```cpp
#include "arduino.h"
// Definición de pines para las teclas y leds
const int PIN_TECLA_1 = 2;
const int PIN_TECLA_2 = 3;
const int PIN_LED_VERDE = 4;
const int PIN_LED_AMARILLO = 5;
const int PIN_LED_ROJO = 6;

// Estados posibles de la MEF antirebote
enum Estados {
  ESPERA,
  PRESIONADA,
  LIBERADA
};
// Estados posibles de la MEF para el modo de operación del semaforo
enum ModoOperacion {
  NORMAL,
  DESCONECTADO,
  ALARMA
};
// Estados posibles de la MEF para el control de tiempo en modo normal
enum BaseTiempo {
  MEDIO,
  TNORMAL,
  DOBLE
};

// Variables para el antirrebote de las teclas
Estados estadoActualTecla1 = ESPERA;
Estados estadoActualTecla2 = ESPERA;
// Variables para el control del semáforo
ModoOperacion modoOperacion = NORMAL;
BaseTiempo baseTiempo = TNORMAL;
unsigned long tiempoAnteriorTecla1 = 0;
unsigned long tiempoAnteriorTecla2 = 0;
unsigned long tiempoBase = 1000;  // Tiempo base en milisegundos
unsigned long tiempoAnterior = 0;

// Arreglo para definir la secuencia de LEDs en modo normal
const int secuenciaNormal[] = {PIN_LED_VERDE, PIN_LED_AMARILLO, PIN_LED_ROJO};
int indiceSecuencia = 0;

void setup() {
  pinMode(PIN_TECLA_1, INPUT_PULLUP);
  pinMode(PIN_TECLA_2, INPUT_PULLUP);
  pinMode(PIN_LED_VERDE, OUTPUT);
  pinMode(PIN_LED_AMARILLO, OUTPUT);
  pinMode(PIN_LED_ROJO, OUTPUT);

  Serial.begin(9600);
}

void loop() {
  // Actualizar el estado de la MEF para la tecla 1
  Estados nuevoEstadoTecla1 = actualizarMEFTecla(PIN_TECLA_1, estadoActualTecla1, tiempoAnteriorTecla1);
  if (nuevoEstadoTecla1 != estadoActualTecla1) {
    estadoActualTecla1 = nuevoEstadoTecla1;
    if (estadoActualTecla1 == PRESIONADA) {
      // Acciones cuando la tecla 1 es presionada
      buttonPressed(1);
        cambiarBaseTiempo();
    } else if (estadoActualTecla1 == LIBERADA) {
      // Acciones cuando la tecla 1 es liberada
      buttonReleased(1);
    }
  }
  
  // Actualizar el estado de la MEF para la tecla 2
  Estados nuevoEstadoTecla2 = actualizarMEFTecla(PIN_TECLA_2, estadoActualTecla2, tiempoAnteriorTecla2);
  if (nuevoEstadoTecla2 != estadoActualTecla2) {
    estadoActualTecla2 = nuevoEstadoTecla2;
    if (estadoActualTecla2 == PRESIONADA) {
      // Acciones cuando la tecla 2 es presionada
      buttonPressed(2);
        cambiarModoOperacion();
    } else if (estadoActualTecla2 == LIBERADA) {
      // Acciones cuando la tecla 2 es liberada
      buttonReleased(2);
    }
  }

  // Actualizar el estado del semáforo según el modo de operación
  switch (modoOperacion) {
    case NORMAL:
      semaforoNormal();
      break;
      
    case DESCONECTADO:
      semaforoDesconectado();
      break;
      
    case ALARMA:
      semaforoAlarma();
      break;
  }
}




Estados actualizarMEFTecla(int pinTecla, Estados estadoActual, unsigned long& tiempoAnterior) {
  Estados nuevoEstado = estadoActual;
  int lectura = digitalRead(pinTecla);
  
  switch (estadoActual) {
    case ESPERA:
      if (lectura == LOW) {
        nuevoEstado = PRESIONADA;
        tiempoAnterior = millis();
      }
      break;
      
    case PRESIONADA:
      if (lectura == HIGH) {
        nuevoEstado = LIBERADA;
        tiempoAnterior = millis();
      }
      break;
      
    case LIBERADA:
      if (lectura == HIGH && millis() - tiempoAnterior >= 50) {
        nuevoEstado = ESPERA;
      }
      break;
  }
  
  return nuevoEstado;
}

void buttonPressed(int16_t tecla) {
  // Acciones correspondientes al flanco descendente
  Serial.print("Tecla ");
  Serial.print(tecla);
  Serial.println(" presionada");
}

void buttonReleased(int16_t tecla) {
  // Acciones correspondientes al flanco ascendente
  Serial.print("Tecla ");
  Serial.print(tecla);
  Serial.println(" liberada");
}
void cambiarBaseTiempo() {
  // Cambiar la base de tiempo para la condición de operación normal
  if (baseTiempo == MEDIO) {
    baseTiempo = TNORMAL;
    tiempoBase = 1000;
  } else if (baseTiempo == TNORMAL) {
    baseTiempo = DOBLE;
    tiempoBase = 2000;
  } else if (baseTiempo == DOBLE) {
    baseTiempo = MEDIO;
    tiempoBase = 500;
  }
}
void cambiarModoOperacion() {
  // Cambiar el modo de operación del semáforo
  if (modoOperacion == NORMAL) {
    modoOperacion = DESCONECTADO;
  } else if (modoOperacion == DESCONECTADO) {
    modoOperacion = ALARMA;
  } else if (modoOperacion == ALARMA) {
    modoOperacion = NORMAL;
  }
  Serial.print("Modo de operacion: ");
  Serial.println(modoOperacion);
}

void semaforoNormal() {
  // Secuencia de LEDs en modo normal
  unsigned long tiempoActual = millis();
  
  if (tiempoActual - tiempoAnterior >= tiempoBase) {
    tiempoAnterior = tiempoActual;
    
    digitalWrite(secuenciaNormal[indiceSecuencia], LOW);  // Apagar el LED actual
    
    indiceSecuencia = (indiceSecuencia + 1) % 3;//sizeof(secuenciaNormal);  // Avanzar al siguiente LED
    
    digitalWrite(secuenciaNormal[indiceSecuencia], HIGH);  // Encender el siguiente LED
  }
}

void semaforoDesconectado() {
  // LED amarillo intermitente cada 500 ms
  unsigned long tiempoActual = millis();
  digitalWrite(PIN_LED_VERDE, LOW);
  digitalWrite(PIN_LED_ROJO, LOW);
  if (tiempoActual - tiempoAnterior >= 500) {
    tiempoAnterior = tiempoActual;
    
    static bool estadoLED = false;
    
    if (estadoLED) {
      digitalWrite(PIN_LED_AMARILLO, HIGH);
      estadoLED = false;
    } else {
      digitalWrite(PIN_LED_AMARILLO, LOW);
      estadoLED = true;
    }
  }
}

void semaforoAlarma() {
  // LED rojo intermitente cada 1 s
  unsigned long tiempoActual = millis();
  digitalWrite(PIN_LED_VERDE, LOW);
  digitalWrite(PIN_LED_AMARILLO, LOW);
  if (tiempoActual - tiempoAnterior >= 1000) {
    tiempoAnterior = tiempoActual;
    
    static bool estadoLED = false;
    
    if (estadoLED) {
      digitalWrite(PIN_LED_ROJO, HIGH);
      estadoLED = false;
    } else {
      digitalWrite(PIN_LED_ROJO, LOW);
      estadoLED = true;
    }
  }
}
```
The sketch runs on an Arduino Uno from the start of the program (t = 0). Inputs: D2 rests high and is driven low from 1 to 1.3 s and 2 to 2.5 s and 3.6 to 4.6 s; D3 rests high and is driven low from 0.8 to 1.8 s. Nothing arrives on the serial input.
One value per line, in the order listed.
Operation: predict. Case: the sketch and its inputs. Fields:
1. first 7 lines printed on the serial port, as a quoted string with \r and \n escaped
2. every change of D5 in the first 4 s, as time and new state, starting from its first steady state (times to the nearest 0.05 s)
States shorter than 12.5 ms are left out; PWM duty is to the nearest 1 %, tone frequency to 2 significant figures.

"Tecla 2 presionada\r\nModo de operacion: 1\r\nTecla 1 presionada\r\nTecla 1 liberada\r\nTecla 2 liberada\r\nTecla 1 presionada\r\nTecla 1 liberada\r\n"
0 s low; 1.3 s high; 1.8 s low; 2.3 s high; 2.8 s low; 3.3 s high; 3.8 s low
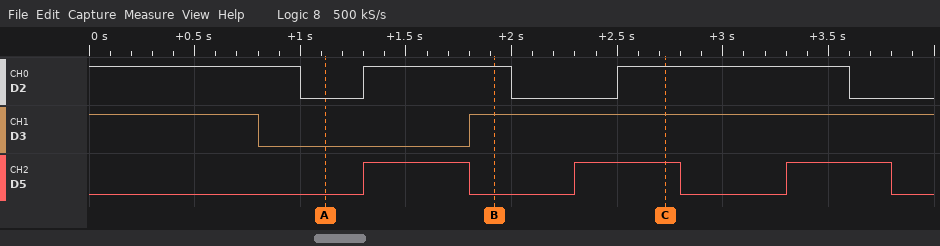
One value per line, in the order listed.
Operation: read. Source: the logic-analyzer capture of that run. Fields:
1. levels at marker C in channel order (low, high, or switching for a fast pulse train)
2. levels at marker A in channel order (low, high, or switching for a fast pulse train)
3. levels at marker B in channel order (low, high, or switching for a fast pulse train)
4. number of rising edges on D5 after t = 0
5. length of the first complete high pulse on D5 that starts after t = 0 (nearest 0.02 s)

D2 high, D3 high, D5 high
D2 low, D3 low, D5 low
D2 high, D3 high, D5 low
3
0.50 s
